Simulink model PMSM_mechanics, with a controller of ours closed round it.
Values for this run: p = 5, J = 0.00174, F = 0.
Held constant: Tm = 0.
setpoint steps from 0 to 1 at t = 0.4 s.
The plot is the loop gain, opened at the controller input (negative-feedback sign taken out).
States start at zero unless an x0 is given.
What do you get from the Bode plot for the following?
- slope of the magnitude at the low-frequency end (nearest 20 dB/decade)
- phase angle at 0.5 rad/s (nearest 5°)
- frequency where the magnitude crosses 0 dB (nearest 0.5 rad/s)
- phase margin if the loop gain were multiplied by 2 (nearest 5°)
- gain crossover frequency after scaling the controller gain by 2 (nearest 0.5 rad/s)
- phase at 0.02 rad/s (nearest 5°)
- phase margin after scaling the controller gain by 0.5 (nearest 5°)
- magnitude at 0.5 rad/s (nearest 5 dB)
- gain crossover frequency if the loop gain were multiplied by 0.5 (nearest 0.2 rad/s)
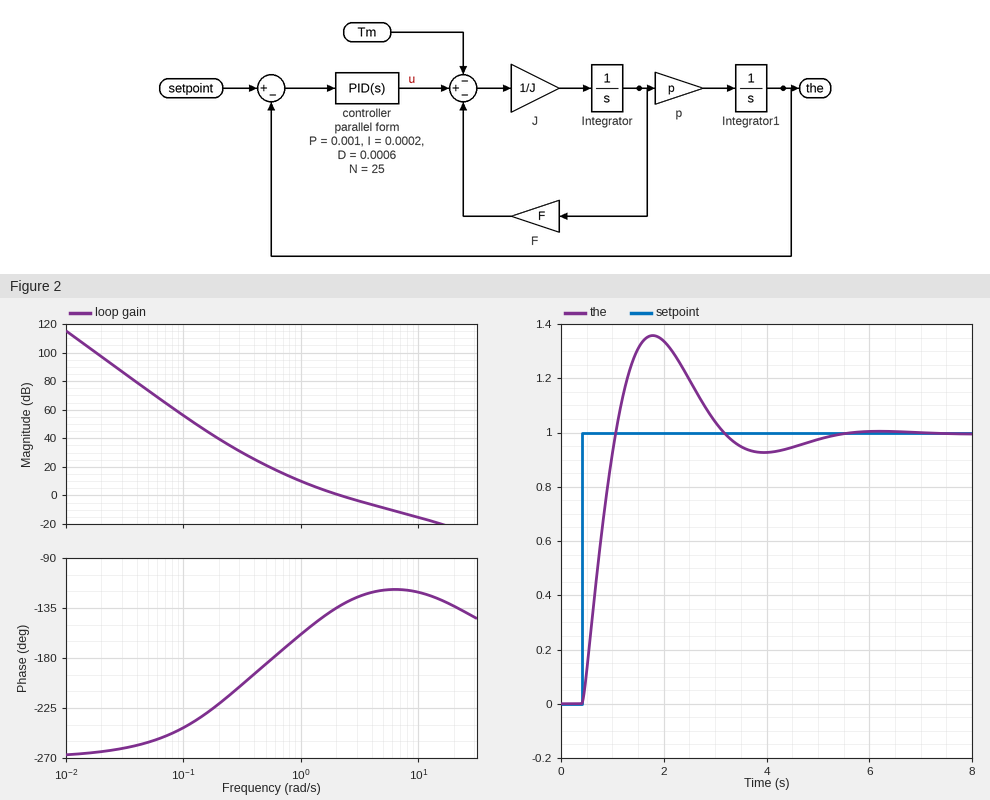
-60 dB/decade
-185°
2.0 rad/s
60°
4.0 rad/s
-265°
30°
20 dB
1.4 rad/s
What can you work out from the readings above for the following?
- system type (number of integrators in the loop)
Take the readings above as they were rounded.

3
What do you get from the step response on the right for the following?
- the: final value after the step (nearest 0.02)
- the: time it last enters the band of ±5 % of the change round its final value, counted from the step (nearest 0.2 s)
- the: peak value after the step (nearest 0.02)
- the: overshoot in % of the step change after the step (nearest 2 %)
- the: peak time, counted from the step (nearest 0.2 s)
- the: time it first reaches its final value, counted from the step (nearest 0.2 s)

1.00
4.2 s
1.36
36 %
1.4 s
0.6 s
